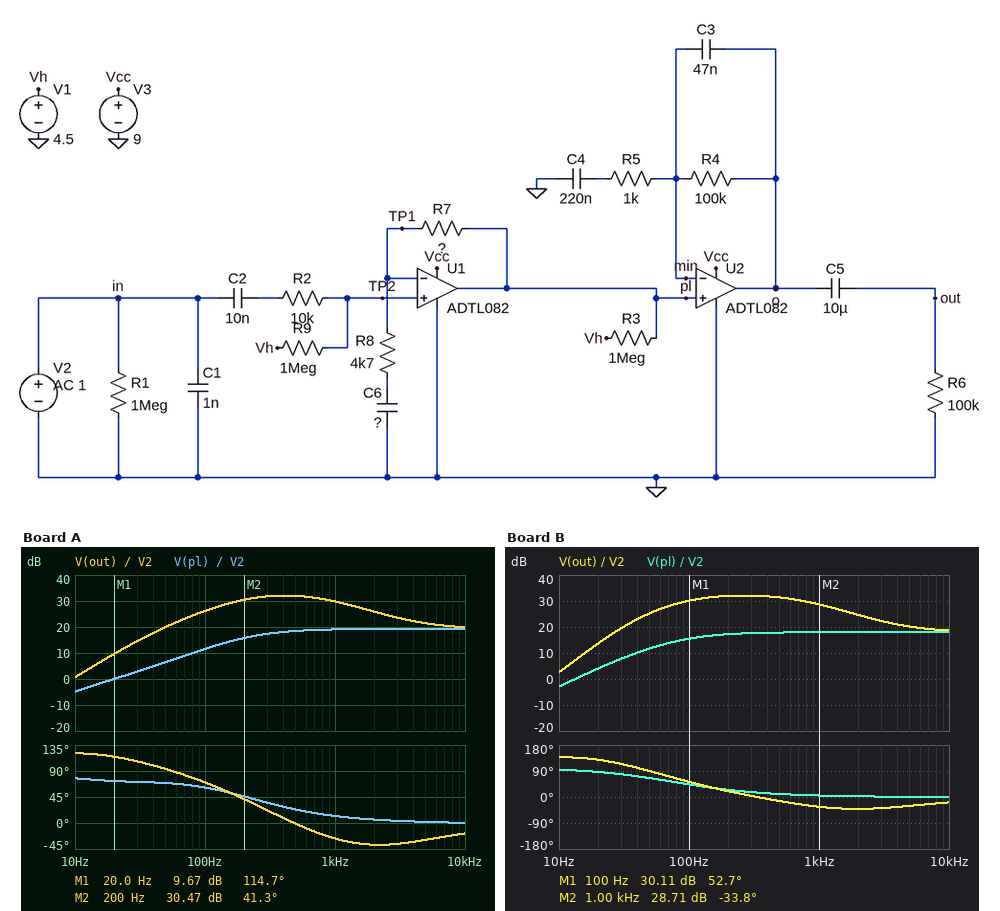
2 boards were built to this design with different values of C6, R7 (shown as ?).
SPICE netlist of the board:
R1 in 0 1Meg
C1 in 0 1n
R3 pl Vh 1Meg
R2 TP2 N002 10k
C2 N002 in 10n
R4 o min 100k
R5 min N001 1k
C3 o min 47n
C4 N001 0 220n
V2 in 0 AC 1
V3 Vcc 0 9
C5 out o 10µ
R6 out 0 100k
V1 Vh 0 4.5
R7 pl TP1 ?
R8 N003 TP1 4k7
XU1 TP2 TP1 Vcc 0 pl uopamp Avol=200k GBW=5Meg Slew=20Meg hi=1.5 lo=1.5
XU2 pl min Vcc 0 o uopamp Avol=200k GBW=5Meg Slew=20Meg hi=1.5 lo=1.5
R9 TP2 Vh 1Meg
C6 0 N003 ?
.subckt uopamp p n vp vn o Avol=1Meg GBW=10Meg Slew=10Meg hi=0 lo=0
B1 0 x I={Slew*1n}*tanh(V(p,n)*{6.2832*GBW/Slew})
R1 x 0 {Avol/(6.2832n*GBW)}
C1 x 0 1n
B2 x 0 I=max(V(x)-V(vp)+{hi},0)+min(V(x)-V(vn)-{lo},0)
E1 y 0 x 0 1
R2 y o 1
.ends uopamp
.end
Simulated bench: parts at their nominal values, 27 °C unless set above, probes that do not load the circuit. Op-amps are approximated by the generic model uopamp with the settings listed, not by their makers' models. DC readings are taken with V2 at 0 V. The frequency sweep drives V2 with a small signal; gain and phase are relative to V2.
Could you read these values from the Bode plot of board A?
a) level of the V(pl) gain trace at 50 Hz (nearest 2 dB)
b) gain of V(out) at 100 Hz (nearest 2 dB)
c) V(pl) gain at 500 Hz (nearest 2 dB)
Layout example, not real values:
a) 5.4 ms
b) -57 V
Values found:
a) 6 dB
b) 26 dB
c) 18 dB
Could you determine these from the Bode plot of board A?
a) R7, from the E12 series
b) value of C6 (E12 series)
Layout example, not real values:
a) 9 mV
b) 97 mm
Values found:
a) 39 kΩ
b) 150 nF
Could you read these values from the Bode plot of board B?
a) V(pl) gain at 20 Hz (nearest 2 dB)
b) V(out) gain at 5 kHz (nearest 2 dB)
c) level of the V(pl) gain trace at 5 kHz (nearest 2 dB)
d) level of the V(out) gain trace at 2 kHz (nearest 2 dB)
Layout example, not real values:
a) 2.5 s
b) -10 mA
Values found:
a) 4 dB
b) 20 dB
c) 18 dB
d) 24 dB
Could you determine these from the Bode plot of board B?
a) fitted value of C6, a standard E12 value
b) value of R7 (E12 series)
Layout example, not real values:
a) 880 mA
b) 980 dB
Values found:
a) 390 nF
b) 33 kΩ
